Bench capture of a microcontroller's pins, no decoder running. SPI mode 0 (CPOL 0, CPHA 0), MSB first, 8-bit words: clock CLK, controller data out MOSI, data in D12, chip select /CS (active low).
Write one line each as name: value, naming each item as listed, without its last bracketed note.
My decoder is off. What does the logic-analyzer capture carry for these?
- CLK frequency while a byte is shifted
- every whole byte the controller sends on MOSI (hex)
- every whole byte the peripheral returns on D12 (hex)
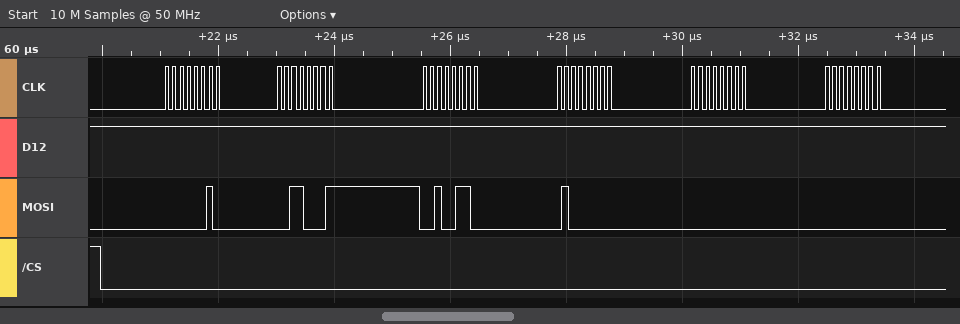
CLK frequency while a byte is shifted: 8 MHz
every whole byte the controller sends on MOSI: 02 31 26 40 00 00
every whole byte the peripheral returns on D12: FF FF FF FF FF FF
